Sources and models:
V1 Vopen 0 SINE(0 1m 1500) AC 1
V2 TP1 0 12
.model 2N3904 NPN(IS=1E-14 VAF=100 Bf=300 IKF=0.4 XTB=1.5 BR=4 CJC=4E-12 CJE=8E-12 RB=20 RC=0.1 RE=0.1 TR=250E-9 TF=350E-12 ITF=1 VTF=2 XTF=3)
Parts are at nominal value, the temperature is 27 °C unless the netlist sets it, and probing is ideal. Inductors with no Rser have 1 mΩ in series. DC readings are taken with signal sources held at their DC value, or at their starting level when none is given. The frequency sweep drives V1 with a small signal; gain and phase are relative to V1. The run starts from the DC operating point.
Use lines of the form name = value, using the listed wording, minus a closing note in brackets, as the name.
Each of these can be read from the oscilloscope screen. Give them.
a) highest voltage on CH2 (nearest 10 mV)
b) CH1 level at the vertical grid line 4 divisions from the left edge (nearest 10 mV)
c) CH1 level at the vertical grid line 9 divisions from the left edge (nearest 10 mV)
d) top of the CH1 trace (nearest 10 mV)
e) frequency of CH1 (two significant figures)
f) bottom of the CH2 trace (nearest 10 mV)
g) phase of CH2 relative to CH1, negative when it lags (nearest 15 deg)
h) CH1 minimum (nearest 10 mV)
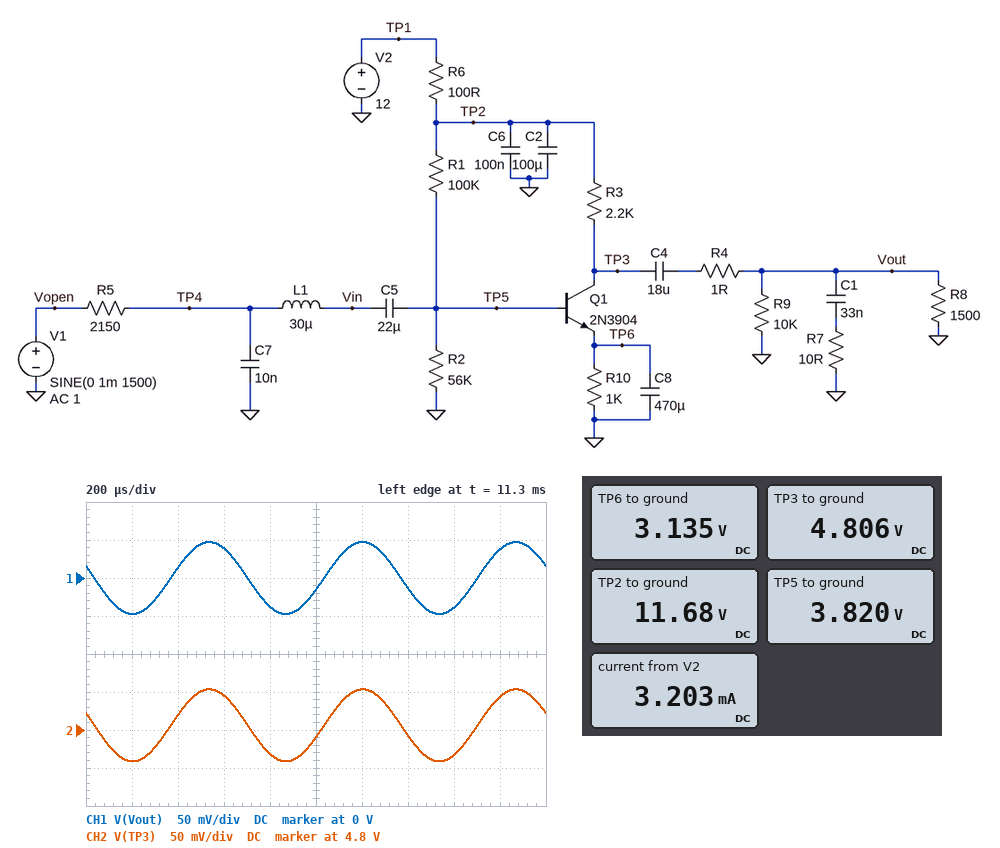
highest voltage on CH2 = 4.85 V
CH1 level at the vertical grid line 4 divisions from the left edge = -40 mV
CH1 level at the vertical grid line 9 divisions from the left edge = 40 mV
top of the CH1 trace = 50 mV
frequency of CH1 = 1.5 kHz
bottom of the CH2 trace = 4.76 V
phase of CH2 relative to CH1, negative when it lags = 0 deg
CH1 minimum = -50 mV
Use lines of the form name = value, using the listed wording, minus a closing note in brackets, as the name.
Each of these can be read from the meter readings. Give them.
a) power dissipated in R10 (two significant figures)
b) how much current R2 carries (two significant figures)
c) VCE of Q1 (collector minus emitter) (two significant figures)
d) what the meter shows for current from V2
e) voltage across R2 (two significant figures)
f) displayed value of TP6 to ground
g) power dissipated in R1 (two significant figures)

power dissipated in R10 = 9.8 mW
how much current R2 carries = 68 µA
VCE of Q1 (collector minus emitter) = 1.7 V
what the meter shows for current from V2 = 3.203 mA
voltage across R2 = 3.8 V
displayed value of TP6 to ground = 3.135 V
power dissipated in R1 = 620 µW
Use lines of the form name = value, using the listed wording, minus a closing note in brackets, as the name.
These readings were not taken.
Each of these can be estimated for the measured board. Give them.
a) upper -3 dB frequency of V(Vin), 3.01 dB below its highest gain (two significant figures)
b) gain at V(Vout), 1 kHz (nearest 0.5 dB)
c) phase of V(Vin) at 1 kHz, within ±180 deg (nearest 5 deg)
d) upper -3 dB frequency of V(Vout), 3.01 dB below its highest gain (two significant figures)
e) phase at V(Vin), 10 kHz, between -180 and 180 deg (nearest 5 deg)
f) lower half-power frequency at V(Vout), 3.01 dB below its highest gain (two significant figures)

upper -3 dB frequency of V(Vin), 3.01 dB below its highest gain = 29 Hz
gain at V(Vout), 1 kHz = 33.5 dB
phase of V(Vin) at 1 kHz, within ±180 deg = -5 deg
upper -3 dB frequency of V(Vout), 3.01 dB below its highest gain = 5.2 kHz
phase at V(Vin), 10 kHz, between -180 and 180 deg = -35 deg
lower half-power frequency at V(Vout), 3.01 dB below its highest gain = 24 Hz
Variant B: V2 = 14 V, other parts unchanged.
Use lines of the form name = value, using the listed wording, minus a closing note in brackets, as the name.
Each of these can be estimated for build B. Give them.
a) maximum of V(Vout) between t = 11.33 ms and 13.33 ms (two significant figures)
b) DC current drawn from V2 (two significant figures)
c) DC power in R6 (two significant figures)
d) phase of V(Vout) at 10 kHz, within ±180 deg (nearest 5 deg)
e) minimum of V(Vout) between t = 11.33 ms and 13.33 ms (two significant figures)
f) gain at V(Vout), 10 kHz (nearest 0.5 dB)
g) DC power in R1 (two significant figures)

maximum of V(Vout) between t = 11.33 ms and 13.33 ms = 52 mV
DC current drawn from V2 = 3.8 mA
DC power in R6 = 1.5 mW
phase of V(Vout) at 10 kHz, within ±180 deg = 90 deg
minimum of V(Vout) between t = 11.33 ms and 13.33 ms = -52 mV
gain at V(Vout), 10 kHz = 27.0 dB
DC power in R1 = 840 µW
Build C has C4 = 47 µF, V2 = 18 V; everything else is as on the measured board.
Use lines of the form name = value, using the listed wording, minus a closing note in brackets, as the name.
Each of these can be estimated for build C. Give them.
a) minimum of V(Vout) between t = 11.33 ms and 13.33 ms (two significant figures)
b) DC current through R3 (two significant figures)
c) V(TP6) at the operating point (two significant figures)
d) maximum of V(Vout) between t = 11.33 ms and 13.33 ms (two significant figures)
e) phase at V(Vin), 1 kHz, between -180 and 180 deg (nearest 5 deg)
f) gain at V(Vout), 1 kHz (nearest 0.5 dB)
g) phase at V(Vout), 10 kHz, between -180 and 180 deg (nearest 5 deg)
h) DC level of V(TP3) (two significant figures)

minimum of V(Vout) between t = 11.33 ms and 13.33 ms = -58 mV
DC current through R3 = 5.0 mA
V(TP6) at the operating point = 5.0 V
maximum of V(Vout) between t = 11.33 ms and 13.33 ms = 58 mV
phase at V(Vin), 1 kHz, between -180 and 180 deg = -5 deg
gain at V(Vout), 1 kHz = 35.5 dB
phase at V(Vout), 10 kHz, between -180 and 180 deg = 95 deg
DC level of V(TP3) = 6.6 V
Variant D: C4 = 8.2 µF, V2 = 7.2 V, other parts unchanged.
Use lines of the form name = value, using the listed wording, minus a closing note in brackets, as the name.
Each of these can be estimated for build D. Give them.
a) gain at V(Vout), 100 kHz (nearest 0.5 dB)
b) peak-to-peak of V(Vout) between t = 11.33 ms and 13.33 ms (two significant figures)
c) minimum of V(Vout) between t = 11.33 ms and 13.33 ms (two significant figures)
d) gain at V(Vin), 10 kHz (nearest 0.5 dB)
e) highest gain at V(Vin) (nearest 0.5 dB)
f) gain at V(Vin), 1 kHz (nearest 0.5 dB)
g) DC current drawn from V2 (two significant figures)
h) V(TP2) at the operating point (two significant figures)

gain at V(Vout), 100 kHz = -13.0 dB
peak-to-peak of V(Vout) between t = 11.33 ms and 13.33 ms = 65 mV
minimum of V(Vout) between t = 11.33 ms and 13.33 ms = -32 mV
gain at V(Vin), 10 kHz = -6.0 dB
highest gain at V(Vin) = 0 dB
gain at V(Vin), 1 kHz = -3.5 dB
DC current drawn from V2 = 1.7 mA
V(TP2) at the operating point = 7.0 V
